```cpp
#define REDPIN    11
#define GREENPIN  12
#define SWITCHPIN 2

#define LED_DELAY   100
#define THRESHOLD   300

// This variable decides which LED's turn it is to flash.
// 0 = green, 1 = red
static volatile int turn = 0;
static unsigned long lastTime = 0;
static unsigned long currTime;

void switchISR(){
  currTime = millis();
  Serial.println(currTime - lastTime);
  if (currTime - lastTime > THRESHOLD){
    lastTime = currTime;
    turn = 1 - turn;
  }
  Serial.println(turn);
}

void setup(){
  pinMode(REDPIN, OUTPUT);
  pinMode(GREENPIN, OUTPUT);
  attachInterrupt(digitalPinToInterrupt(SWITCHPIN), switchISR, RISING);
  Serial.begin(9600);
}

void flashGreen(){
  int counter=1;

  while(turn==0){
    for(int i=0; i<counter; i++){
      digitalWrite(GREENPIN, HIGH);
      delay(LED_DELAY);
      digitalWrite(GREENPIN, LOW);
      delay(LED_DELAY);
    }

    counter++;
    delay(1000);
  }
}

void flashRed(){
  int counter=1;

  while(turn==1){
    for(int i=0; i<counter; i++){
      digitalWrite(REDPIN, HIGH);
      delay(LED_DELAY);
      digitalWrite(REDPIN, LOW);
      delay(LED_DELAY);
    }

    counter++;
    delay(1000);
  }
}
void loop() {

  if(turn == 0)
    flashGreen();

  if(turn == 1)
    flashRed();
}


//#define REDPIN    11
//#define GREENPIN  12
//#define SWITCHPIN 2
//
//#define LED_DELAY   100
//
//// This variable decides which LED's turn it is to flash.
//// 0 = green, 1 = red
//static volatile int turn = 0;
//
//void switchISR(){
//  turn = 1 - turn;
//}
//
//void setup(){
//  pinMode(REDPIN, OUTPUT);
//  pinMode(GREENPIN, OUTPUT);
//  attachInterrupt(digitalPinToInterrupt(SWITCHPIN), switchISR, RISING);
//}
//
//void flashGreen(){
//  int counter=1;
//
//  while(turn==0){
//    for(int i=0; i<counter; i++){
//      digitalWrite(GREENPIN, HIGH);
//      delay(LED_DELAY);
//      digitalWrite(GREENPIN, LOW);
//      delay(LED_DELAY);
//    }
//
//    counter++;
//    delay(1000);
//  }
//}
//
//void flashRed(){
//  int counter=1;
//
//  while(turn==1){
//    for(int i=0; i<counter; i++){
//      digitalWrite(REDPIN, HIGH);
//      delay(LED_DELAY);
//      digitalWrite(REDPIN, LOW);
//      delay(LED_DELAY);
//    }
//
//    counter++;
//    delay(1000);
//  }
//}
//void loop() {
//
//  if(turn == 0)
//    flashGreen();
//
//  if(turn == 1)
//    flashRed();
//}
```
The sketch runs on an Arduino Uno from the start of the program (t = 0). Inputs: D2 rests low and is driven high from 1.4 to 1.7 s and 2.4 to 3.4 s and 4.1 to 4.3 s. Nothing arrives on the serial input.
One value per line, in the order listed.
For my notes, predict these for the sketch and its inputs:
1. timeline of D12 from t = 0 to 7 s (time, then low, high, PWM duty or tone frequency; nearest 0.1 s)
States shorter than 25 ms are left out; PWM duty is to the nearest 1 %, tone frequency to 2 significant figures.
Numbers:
0 s high; 0.1 s low; 1.2 s high; 1.3 s low; 1.4 s high; 1.5 s low; 2.6 s high; 2.7 s low; 2.8 s high; 2.9 s low; 3 s high; 3.1 s low
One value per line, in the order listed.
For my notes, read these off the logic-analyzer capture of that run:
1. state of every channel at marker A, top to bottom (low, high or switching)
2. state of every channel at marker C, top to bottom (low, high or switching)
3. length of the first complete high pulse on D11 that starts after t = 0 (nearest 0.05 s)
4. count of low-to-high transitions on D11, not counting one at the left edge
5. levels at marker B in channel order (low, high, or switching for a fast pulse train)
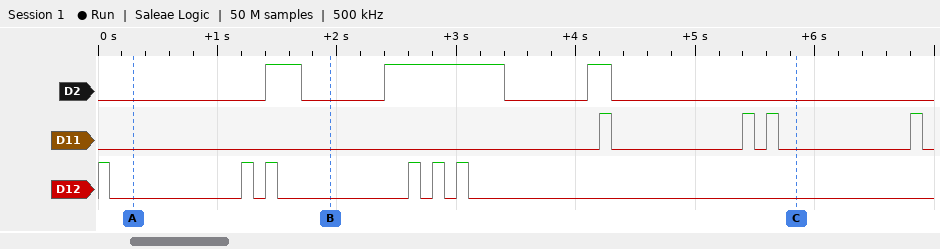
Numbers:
D2 low, D11 low, D12 low
D2 low, D11 low, D12 low
0.10 s
4
D2 low, D11 low, D12 low
